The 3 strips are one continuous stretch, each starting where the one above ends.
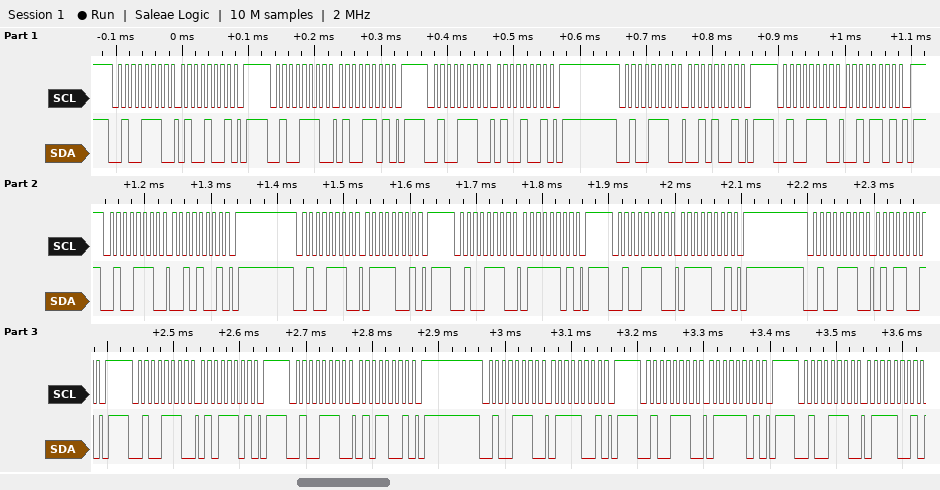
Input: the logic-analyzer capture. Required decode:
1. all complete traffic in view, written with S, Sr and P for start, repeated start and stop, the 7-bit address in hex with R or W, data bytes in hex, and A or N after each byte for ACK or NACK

S 27W A 49 A P S 27W A 4D A P S 27W A 49 A P S 27W A 29 A P S 27W A 2D A P S 27W A 29 A P S 27W A 79 A P S 27W A 7D A P S 27W A 79 A P S 27W A 59 A P S 27W A 5D A P S 27W A 59 A P S 27W A 79 A P S 27W A 7D A P S 27W A 79 A
